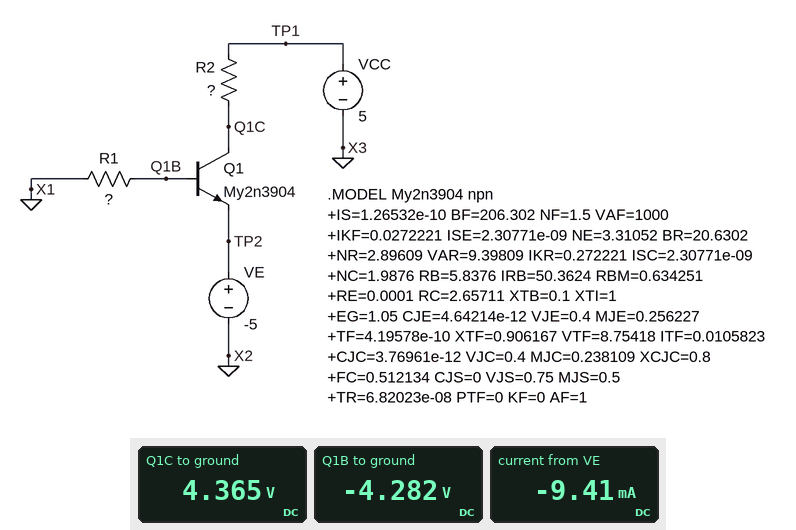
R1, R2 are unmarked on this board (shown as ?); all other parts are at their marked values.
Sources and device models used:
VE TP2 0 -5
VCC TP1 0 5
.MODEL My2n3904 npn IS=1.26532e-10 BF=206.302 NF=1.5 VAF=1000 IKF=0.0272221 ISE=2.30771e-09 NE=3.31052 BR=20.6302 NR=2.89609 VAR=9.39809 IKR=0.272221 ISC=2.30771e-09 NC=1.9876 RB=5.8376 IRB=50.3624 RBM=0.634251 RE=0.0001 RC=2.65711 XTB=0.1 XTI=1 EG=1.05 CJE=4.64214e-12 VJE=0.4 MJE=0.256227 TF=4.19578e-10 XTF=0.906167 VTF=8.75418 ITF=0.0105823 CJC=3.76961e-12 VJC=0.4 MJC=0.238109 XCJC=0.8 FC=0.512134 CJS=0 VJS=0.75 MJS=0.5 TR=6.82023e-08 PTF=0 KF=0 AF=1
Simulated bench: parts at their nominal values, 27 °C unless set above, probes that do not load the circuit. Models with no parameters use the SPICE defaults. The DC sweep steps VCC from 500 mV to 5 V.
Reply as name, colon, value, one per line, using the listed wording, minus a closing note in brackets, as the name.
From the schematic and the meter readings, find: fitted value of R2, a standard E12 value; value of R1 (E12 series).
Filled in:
fitted value of R2, a standard E12 value: 68 Ω
value of R1: 56 kΩ
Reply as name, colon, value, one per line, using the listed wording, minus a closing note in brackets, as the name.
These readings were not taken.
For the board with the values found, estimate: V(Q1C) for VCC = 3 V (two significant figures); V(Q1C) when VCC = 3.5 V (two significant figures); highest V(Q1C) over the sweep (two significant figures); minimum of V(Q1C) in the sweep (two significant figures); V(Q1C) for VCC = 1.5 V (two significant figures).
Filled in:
V(Q1C) for VCC = 3 V: 2.4 V
V(Q1C) when VCC = 3.5 V: 2.9 V
highest V(Q1C) over the sweep: 4.4 V
minimum of V(Q1C) in the sweep: -130 mV
V(Q1C) for VCC = 1.5 V: 870 mV
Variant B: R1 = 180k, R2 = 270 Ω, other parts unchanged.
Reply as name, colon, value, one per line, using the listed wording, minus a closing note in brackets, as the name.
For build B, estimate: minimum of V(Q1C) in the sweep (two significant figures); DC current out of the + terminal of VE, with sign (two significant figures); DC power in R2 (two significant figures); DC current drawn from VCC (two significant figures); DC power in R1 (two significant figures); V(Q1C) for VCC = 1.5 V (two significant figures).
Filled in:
minimum of V(Q1C) in the sweep: -350 mV
DC current out of the + terminal of VE, with sign: -3.2 mA
DC power in R2: 2.7 mW
DC current drawn from VCC: 3.2 mA
DC power in R1: 100 µW
V(Q1C) for VCC = 1.5 V: 650 mV
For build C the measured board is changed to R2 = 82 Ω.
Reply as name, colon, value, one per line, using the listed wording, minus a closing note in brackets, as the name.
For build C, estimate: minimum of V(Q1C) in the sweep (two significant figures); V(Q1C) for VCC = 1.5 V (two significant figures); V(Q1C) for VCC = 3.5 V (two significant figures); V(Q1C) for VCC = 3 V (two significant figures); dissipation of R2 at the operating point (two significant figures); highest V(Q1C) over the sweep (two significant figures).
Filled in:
minimum of V(Q1C) in the sweep: -260 mV
V(Q1C) for VCC = 1.5 V: 740 mV
V(Q1C) for VCC = 3.5 V: 2.7 V
V(Q1C) for VCC = 3 V: 2.2 V
dissipation of R2 at the operating point: 7.1 mW
highest V(Q1C) over the sweep: 4.2 V
